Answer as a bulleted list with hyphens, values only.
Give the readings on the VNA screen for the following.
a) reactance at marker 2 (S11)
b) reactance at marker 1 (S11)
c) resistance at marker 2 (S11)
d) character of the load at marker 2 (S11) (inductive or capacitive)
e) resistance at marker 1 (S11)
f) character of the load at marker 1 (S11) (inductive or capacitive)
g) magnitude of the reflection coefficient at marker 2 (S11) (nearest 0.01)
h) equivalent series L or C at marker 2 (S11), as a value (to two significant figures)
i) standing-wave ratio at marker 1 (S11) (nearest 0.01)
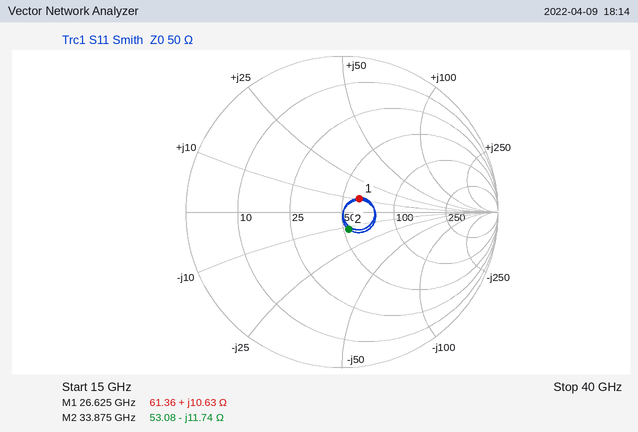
- -11.74 Ω
- +10.63 Ω
- 53.08 Ω
- capacitive
- 61.36 Ω
- inductive
- 0.12
- 400 fF
- 1.32
